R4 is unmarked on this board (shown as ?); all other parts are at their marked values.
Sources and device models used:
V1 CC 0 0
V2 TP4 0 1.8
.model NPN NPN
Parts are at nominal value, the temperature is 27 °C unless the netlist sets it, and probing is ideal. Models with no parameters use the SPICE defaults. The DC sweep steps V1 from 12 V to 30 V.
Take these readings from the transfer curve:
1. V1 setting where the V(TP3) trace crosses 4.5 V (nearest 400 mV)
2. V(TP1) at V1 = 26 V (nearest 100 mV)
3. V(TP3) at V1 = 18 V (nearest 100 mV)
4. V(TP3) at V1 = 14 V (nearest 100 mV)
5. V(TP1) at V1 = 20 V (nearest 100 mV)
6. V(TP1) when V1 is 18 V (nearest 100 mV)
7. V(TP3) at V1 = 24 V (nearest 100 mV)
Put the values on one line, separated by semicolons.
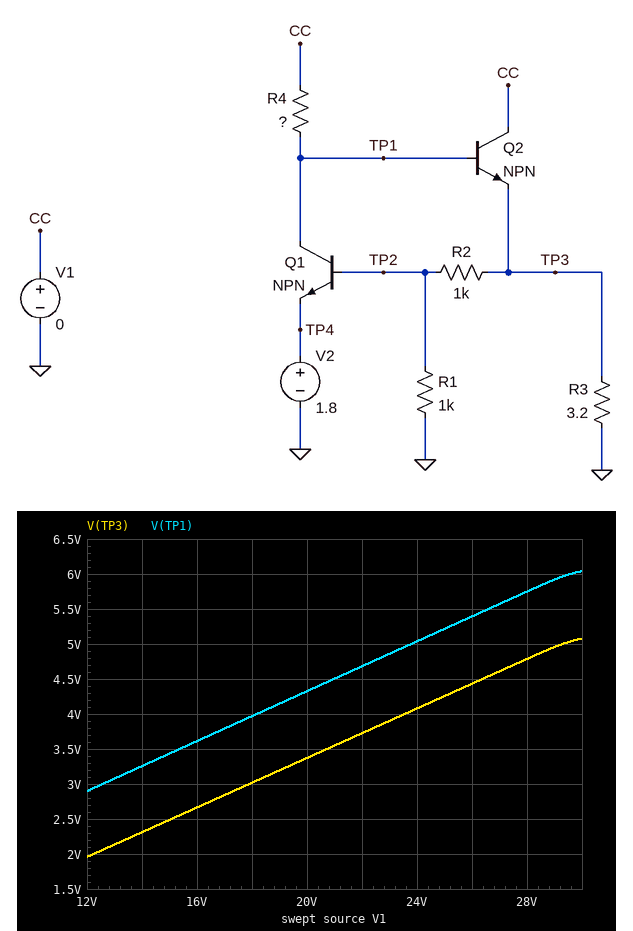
26.4 V; 5.4 V; 3.0 V; 2.3 V; 4.3 V; 4.0 V; 4.1 V
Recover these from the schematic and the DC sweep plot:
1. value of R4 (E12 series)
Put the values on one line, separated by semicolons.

1.5 kΩ
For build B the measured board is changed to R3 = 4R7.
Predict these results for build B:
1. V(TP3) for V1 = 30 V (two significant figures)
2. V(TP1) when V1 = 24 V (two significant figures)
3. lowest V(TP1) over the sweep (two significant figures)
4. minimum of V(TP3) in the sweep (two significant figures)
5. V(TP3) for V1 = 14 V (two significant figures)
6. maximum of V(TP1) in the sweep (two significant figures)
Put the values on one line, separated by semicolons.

5.3 V; 6.1 V; 3.6 V; 2.7 V; 3.1 V; 6.2 V
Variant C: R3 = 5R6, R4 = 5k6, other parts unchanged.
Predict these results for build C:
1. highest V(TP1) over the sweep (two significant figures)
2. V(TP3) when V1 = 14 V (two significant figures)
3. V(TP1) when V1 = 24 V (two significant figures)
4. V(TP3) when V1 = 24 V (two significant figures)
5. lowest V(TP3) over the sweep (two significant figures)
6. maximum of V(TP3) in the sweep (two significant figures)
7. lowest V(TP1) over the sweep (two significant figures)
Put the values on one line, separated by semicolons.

3.6 V; 1.2 V; 3.0 V; 2.1 V; 1.0 V; 2.7 V; 1.9 V
